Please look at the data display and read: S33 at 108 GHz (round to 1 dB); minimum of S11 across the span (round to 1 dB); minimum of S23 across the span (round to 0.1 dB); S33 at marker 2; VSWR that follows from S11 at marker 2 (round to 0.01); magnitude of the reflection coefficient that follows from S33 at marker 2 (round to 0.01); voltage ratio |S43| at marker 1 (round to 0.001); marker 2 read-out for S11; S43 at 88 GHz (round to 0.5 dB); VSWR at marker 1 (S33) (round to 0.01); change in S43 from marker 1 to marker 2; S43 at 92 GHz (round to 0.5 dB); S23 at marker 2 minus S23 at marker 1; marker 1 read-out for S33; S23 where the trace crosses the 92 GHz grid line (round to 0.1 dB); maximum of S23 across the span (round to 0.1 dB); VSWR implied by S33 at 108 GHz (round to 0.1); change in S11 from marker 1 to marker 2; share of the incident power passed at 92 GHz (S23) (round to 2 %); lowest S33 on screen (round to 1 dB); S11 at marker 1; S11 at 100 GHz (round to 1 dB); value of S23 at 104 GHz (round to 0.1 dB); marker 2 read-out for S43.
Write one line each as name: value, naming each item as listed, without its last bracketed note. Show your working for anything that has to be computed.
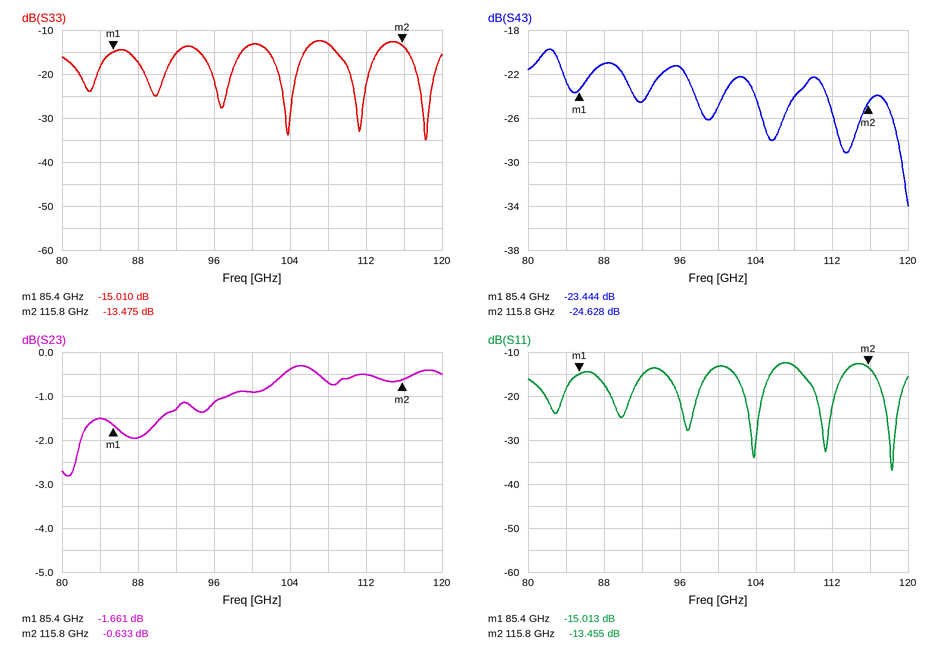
S33 at 108 GHz: -13 dB
minimum of S11 across the span: -37 dB
minimum of S23 across the span: -2.8 dB
S33 at marker 2: -13.475 dB
VSWR that follows from S11 at marker 2: (1 + 0.2124)/(1 − 0.2124) ≈ 1.54
magnitude of the reflection coefficient that follows from S33 at marker 2: 10^(-13.475/20) ≈ 0.21
voltage ratio |S43| at marker 1: 10^(-23.444/20) ≈ 0.067
marker 2 read-out for S11: -13.455 dB
S43 at 88 GHz: -21.0 dB
VSWR at marker 1 (S33): (1 + 0.1776)/(1 − 0.1776) ≈ 1.43
change in S43 from marker 1 to marker 2: -24.628 − (-23.444) = -1.184 dB
S43 at 92 GHz: -24.5 dB
S23 at marker 2 minus S23 at marker 1: -0.633 − (-1.661) = 1.028 dB
marker 1 read-out for S33: -15.010 dB
S23 where the trace crosses the 92 GHz grid line: -1.3 dB
maximum of S23 across the span: -0.3 dB
VSWR implied by S33 at 108 GHz: |Γ| = 10^(-13/20) = 0.2239; VSWR = (1 + 0.2239)/(1 − 0.2239) ≈ 1.6
change in S11 from marker 1 to marker 2: -13.455 − (-15.013) = 1.558 dB
share of the incident power passed at 92 GHz (S23): 10^(-1.3/10) ≈ 74 %
lowest S33 on screen: -35 dB
S11 at marker 1: -15.013 dB
S11 at 100 GHz: -13 dB
value of S23 at 104 GHz: -0.4 dB
marker 2 read-out for S43: -24.628 dB
